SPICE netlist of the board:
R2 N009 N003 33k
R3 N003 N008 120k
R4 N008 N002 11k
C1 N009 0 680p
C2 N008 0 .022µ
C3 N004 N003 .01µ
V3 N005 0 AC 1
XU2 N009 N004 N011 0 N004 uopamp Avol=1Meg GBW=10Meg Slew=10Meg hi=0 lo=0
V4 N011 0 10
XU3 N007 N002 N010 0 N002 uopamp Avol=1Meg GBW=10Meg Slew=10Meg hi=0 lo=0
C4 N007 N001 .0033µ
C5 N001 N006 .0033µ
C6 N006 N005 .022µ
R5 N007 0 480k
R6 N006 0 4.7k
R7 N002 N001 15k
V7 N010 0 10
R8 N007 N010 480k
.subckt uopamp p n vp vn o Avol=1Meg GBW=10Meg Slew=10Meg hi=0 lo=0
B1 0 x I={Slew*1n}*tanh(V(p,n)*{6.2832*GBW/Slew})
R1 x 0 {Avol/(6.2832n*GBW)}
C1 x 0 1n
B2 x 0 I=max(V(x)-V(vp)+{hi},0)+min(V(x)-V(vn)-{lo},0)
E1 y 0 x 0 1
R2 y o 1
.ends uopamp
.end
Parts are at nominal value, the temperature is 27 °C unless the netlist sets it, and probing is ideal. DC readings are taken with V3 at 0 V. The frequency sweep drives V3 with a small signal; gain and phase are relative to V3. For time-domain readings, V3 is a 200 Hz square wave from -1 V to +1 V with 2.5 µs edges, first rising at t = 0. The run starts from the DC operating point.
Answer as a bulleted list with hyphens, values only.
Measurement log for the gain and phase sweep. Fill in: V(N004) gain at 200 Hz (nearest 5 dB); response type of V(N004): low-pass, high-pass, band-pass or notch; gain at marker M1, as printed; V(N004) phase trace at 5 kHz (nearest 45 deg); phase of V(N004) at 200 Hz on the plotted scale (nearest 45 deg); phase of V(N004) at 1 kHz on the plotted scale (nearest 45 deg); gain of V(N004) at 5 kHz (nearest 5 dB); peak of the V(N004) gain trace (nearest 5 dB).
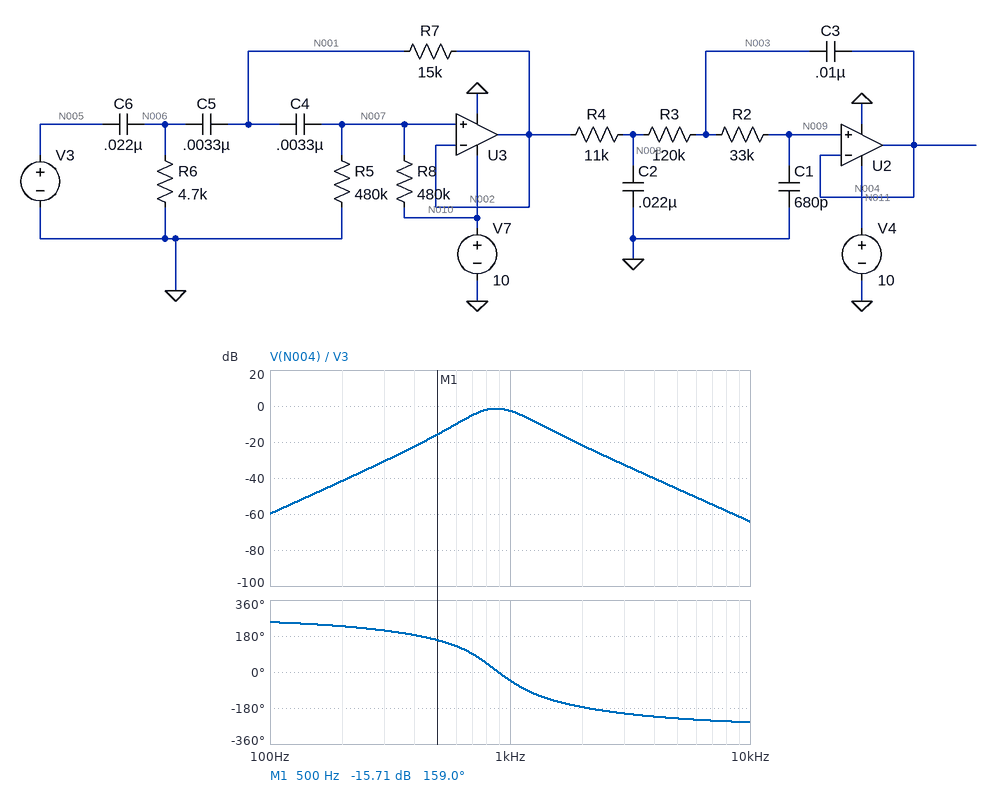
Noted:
- -40 dB
- band-pass
- -15.71 dB
- -225 deg
- 225 deg
- -45 deg
- -45 dB
- 0 dB
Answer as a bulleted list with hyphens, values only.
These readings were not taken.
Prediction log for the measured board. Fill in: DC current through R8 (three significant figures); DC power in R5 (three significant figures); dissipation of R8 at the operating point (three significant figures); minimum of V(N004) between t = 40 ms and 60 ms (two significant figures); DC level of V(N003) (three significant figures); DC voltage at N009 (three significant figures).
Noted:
- 10.4 µA
- 52.1 µW
- 52.1 µW
- 4.7 V
- 5.00 V
- 5.00 V
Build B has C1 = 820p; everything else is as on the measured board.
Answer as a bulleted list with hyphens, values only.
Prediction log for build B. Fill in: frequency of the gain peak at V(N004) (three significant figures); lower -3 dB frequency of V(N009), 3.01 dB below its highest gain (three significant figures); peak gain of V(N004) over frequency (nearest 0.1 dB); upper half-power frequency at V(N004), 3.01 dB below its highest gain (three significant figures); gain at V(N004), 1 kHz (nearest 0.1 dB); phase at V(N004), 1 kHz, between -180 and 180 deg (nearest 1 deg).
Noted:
- 842 Hz
- 690 Hz
- -2.6 dB
- 1.04 kHz
- -4.7 dB
- -55 deg
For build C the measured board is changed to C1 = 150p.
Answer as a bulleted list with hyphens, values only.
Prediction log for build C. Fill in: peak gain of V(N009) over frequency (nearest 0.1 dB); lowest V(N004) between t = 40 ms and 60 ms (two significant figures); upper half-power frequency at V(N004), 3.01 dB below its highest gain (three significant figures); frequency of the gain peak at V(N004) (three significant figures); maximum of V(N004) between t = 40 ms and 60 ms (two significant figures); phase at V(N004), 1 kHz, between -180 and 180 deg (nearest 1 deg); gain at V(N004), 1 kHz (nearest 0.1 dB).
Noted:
- -0.9 dB
- 4.4 V
- 2.25 kHz
- 1.95 kHz
- 5.6 V
- 42 deg
- -3.4 dB
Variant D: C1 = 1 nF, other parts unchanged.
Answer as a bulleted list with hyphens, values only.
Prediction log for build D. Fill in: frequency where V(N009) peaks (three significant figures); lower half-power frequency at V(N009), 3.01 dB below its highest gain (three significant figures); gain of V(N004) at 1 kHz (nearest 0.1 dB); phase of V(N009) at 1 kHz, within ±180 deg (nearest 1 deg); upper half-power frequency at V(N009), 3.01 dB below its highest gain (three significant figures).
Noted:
- 814 Hz
- 662 Hz
- -7.1 dB
- -65 deg
- 1.01 kHz
